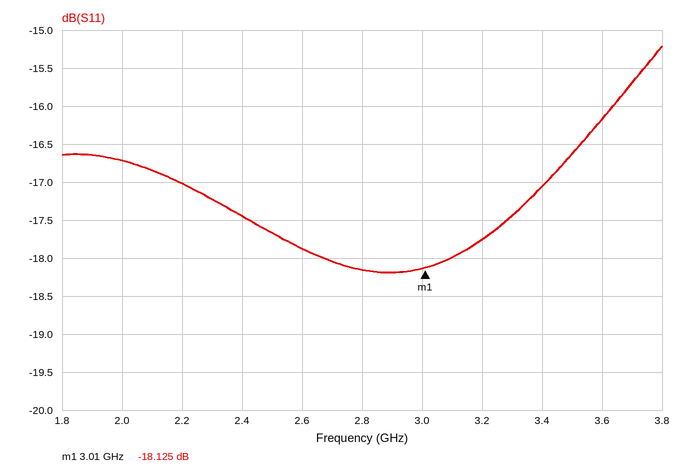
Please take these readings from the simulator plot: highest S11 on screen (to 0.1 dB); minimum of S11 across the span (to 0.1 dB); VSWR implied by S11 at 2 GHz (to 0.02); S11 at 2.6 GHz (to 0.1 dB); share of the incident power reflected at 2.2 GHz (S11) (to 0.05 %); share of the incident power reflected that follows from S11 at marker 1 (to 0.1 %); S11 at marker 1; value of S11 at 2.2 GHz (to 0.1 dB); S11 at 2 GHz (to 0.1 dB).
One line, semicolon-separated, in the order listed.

-15.2 dB; -18.2 dB; 1.34; -17.9 dB; 2.00 %; 1.5 %; -18.125 dB; -17.0 dB; -16.7 dB
